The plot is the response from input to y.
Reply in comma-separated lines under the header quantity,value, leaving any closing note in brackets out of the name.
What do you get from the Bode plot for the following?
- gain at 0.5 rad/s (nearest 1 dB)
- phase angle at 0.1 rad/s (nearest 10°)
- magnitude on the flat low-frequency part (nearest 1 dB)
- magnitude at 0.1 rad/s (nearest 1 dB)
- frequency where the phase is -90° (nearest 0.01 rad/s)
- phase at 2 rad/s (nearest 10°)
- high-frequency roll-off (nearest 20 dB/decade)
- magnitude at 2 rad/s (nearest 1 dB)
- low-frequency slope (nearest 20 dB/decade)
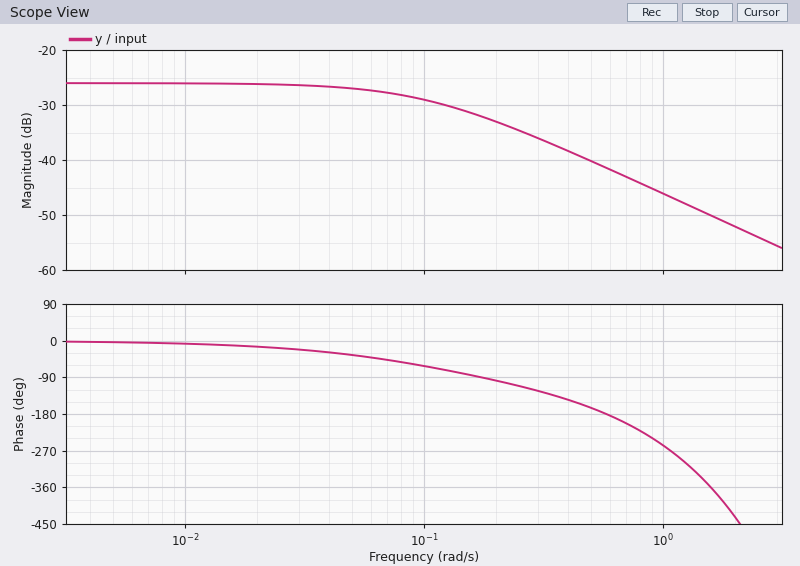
quantity,value
gain at 0.5 rad/s,-40 dB
phase angle at 0.1 rad/s,-60°
magnitude on the flat low-frequency part,-26 dB
magnitude at 0.1 rad/s,-29 dB
frequency where the phase is -90°,0.17 rad/s
phase at 2 rad/s,-430°
high-frequency roll-off,-20 dB/decade
magnitude at 2 rad/s,-52 dB
low-frequency slope,0 dB/decade
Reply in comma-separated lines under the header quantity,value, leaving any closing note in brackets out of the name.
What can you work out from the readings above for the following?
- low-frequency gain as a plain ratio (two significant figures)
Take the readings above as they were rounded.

quantity,value
low-frequency gain as a plain ratio,0.050
